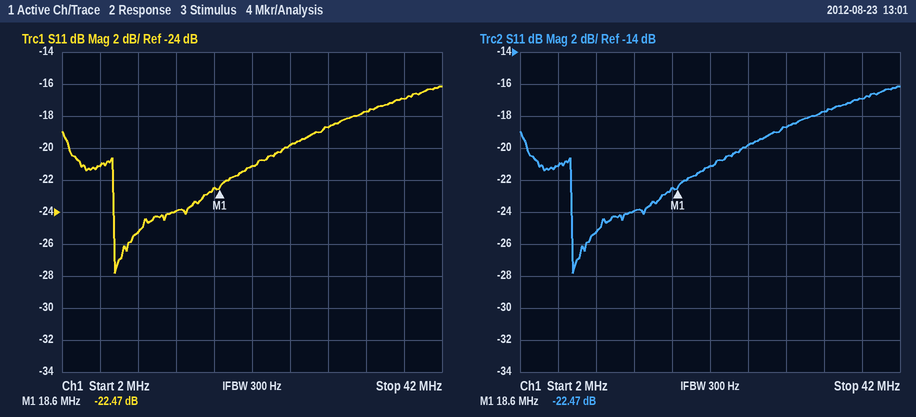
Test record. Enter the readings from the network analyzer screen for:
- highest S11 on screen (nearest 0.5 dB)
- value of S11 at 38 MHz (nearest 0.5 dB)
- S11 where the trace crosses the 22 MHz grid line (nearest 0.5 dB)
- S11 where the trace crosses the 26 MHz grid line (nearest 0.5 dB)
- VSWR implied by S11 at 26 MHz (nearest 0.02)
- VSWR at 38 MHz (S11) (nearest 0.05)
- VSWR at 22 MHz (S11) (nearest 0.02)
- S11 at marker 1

-16.0 dB
-17.0 dB
-21.0 dB
-20.0 dB
1.22
1.35
1.20
-22.47 dB
